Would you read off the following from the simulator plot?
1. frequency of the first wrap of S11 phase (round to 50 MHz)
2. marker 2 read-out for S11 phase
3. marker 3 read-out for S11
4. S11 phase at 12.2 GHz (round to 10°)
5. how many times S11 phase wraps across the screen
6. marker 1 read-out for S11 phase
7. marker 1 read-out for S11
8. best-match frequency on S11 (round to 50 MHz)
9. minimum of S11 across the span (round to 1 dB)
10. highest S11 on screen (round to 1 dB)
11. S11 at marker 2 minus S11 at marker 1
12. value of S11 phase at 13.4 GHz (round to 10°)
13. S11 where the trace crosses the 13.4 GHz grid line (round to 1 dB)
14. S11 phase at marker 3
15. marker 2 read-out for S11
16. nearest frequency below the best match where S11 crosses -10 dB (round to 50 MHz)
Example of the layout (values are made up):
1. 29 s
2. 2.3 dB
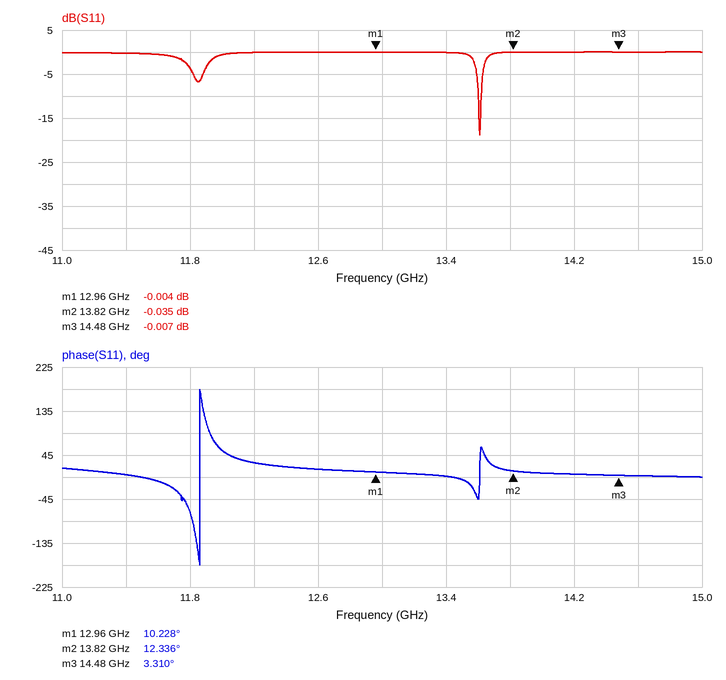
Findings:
1. 11.85 GHz
2. 12.336°
3. -0.007 dB
4. 30°
5. 1
6. 10.228°
7. -0.004 dB
8. 13.60 GHz
9. -19 dB
10. 0 dB
11. -0.031 dB
12. 0°
13. 0 dB
14. 3.310°
15. -0.035 dB
16. 13.60 GHz
